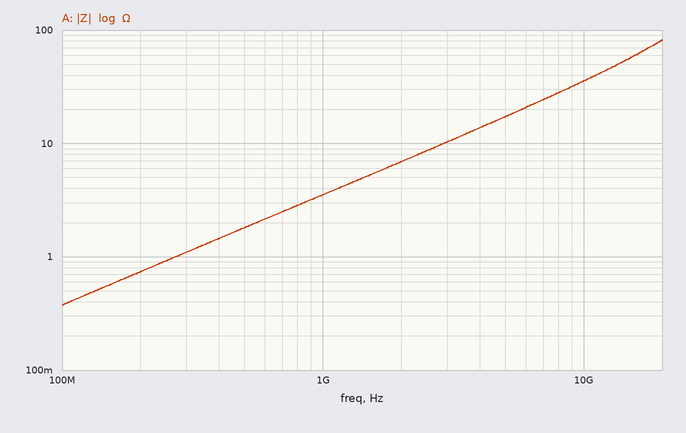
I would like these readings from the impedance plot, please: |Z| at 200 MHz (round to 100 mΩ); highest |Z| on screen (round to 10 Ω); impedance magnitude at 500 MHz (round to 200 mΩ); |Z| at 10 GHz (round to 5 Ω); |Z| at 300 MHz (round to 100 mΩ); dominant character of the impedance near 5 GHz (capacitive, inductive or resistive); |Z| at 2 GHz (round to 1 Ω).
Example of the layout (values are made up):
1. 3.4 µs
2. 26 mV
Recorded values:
1. 700 mΩ
2. 80 Ω
3. 1.8 Ω
4. 35 Ω
5. 1.1 Ω
6. inductive
7. 7 Ω
